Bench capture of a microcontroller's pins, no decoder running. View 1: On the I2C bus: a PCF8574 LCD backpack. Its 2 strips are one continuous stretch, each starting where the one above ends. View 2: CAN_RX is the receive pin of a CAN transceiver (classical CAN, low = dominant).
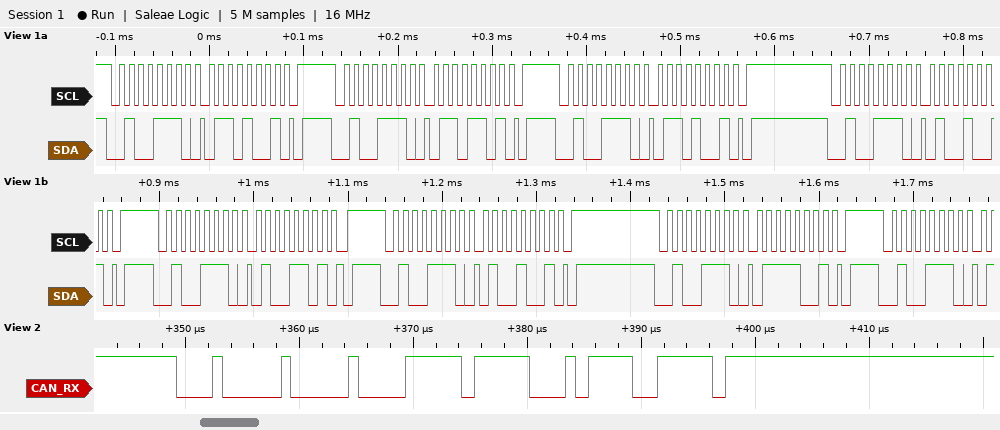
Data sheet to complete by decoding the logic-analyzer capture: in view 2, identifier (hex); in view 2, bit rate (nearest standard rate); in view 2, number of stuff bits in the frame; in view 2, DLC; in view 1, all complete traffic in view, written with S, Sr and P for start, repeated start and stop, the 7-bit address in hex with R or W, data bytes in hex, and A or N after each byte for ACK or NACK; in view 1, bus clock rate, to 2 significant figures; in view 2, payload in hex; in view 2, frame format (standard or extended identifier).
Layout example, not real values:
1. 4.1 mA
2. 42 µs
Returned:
1. 0x100
2. 1000 kbit/s
3. 4
4. 1
5. S 27W A 69 A P S 27W A 6D A P S 27W A 69 A P S 27W A 49 A P S 27W A 4D A P S 27W A 49 A P S 27W A 79 A P S 27W A
6. 100 kHz
7. FF
8. standard
